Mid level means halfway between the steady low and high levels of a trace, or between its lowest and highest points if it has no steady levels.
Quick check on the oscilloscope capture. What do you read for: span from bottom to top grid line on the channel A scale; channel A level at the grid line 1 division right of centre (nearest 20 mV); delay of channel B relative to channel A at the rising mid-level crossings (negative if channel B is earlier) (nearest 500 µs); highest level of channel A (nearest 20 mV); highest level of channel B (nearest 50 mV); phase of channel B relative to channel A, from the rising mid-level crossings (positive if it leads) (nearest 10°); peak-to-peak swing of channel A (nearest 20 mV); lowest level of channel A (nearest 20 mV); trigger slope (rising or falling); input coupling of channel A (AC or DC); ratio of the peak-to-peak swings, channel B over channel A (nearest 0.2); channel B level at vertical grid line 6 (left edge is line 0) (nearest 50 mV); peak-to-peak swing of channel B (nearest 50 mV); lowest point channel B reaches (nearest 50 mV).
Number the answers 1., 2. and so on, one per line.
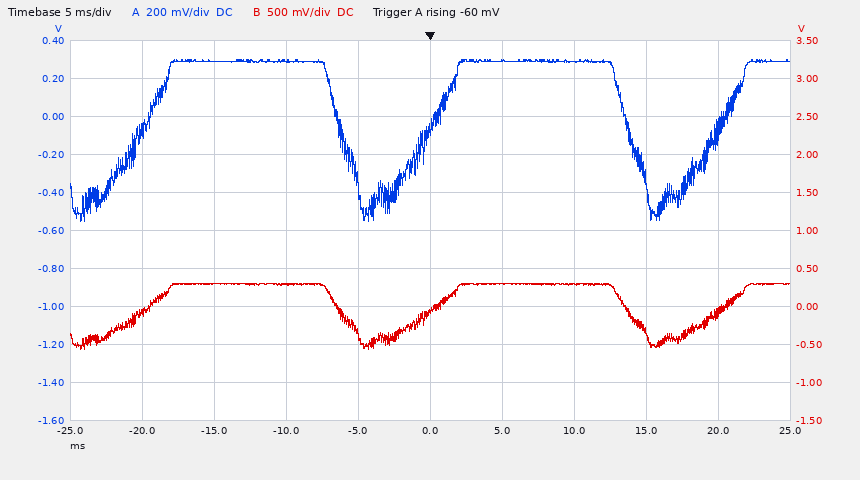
1. 2 V
2. 300 mV
3. 0.0 ms
4. 300 mV
5. 300 mV
6. 0°
7. 860 mV
8. -560 mV
9. rising
10. DC
11. 1.0
12. 300 mV
13. 850 mV
14. -550 mV
